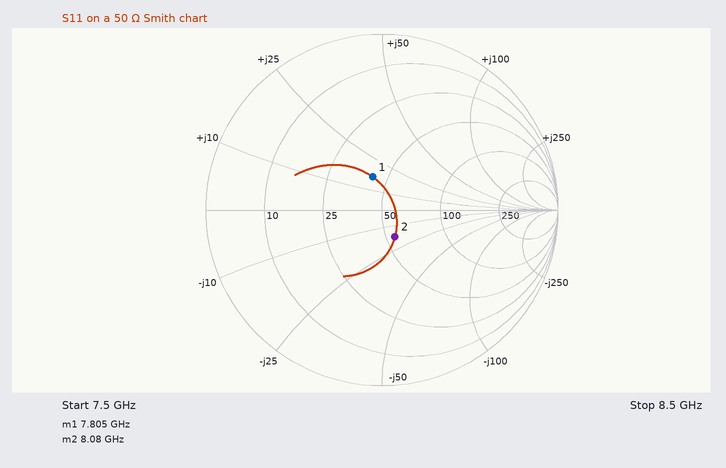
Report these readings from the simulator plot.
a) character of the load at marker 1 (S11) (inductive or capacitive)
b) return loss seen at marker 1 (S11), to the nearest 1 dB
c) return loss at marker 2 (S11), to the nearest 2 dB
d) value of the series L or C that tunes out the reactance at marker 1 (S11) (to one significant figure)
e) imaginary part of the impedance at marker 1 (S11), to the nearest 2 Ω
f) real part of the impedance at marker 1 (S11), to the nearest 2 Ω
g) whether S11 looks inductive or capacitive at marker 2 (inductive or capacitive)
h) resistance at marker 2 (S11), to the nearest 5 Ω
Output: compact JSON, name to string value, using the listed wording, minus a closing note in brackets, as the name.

{"character of the load at marker 1 (S11)": "inductive", "return loss seen at marker 1 (S11), to the nearest 1 dB": "14 dB", "return loss at marker 2 (S11), to the nearest 2 dB": "16 dB", "value of the series L or C that tunes out the reactance at marker 1 (S11)": "1 pF", "imaginary part of the impedance at marker 1 (S11), to the nearest 2 Ω": "+16 Ω", "real part of the impedance at marker 1 (S11), to the nearest 2 Ω": "42 Ω", "whether S11 looks inductive or capacitive at marker 2": "capacitive", "resistance at marker 2 (S11), to the nearest 5 Ω": "55 Ω"}
